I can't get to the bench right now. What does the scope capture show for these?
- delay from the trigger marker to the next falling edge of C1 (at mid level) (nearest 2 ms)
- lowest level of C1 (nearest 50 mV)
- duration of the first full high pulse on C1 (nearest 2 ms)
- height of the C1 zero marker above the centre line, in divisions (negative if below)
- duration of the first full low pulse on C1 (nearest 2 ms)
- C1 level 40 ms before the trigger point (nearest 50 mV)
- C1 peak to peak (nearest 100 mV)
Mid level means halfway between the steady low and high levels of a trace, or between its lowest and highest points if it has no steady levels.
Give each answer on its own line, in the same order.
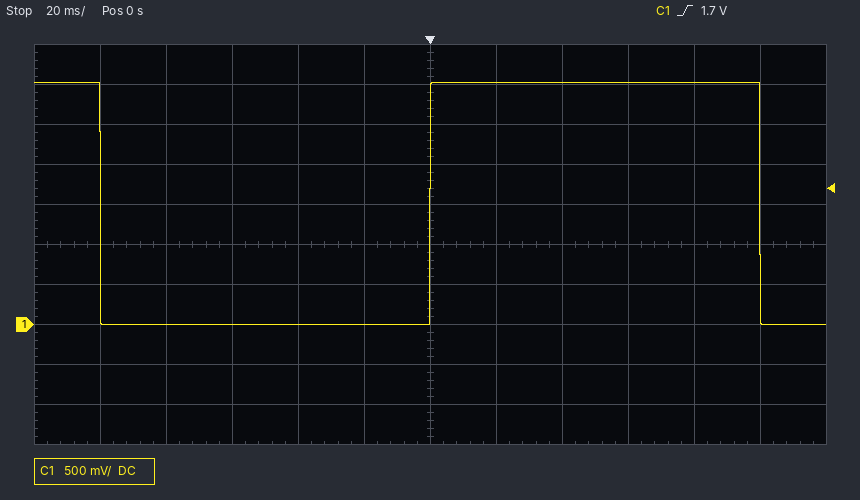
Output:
100 ms
0 mV
100 ms
-2.0 div
100 ms
0 mV
3.00 V
